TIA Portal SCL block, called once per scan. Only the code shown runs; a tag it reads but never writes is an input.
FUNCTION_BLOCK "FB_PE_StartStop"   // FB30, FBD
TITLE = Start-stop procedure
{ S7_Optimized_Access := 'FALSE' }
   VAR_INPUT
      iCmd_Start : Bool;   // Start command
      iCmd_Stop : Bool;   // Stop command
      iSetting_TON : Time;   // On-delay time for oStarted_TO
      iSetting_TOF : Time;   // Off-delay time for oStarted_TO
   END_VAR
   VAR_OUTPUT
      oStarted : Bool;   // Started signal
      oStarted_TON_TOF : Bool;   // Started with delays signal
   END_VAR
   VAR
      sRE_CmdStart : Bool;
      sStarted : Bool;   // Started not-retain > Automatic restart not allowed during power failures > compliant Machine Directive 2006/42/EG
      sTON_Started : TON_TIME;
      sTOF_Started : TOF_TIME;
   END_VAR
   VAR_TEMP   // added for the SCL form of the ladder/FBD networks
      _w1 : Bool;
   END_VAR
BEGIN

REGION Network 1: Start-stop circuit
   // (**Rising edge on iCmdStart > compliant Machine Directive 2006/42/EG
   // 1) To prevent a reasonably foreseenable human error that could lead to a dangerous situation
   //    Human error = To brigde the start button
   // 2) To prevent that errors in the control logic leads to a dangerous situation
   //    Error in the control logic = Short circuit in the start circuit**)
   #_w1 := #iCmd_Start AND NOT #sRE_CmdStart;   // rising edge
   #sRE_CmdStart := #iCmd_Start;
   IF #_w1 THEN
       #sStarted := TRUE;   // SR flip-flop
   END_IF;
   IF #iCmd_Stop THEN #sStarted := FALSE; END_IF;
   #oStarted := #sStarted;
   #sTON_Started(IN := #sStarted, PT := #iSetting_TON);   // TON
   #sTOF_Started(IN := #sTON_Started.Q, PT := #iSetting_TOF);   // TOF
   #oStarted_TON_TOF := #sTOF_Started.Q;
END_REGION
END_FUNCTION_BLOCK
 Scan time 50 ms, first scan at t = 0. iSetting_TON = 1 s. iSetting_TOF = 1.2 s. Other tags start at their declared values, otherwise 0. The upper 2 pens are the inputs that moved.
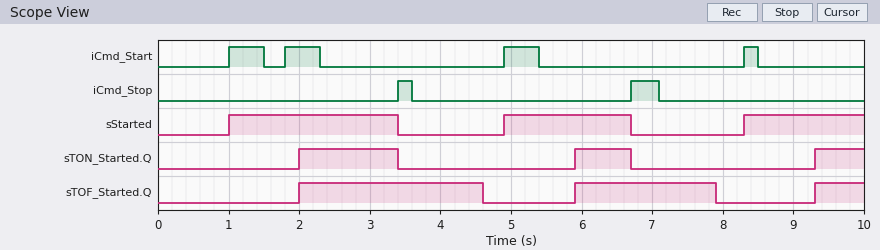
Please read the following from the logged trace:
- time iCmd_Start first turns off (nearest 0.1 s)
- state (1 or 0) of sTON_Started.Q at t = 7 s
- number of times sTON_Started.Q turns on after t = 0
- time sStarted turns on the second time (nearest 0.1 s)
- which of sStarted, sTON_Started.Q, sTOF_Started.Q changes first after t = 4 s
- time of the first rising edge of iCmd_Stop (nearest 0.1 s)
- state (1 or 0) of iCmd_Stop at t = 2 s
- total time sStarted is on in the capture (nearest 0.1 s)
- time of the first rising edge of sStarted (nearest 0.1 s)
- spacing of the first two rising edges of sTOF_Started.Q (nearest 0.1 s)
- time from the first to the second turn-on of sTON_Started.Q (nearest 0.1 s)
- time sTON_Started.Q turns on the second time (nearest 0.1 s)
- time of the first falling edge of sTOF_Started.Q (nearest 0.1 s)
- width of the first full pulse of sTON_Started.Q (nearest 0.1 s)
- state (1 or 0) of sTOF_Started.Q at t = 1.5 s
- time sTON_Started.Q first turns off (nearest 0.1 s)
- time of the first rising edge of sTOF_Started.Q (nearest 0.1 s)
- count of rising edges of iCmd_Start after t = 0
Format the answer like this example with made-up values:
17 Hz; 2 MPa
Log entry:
1.5 s; 0; 3; 4.9 s; sTOF_Started.Q; 3.4 s; 0; 5.9 s; 1.0 s; 3.9 s; 3.9 s; 5.9 s; 4.6 s; 1.4 s; 0; 3.4 s; 2.0 s; 4
